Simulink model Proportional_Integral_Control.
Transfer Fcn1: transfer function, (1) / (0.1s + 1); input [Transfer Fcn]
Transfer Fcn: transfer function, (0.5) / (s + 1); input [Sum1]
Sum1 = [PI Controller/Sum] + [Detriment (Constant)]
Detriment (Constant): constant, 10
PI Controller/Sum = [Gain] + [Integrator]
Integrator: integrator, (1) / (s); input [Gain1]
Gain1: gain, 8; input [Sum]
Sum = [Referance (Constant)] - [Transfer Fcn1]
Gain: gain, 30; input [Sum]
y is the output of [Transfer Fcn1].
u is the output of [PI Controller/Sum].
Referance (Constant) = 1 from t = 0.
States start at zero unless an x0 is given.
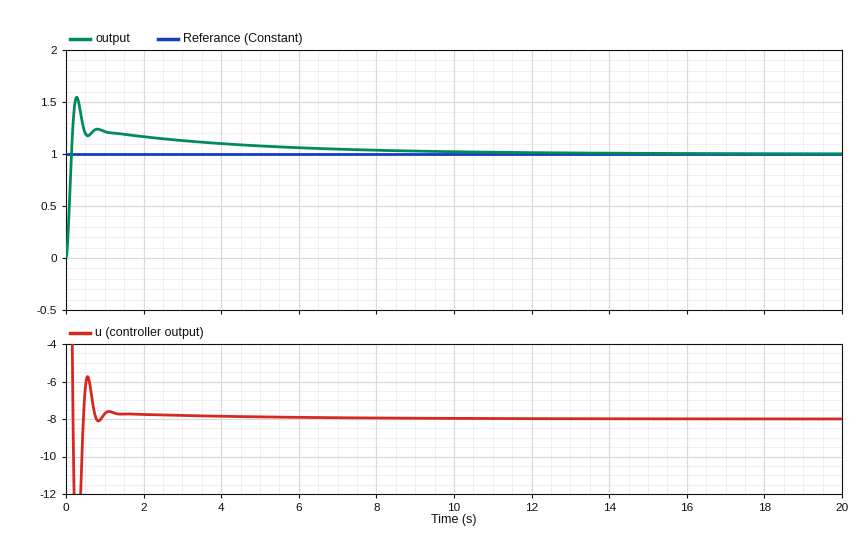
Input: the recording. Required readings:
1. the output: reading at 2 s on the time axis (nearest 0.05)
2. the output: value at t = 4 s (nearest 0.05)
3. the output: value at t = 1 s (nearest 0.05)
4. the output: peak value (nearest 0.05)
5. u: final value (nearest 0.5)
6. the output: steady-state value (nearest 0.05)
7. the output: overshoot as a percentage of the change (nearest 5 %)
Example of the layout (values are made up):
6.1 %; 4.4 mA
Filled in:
1.15; 1.10; 1.20; 1.55; -8.0; 1.00; 55 %
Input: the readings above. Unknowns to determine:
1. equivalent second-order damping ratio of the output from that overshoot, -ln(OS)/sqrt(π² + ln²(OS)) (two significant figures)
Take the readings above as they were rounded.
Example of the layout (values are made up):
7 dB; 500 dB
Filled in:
0.19
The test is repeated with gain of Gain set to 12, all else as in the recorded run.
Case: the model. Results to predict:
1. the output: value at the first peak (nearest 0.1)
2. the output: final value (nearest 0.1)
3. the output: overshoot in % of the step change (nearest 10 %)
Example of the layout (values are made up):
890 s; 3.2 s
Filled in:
1.7; 1.0; 70 %
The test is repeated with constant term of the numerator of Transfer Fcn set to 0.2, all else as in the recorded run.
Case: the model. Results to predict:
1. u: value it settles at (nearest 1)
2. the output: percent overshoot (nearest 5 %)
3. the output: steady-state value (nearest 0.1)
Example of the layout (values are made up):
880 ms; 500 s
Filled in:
-5; 25 %; 1.0
